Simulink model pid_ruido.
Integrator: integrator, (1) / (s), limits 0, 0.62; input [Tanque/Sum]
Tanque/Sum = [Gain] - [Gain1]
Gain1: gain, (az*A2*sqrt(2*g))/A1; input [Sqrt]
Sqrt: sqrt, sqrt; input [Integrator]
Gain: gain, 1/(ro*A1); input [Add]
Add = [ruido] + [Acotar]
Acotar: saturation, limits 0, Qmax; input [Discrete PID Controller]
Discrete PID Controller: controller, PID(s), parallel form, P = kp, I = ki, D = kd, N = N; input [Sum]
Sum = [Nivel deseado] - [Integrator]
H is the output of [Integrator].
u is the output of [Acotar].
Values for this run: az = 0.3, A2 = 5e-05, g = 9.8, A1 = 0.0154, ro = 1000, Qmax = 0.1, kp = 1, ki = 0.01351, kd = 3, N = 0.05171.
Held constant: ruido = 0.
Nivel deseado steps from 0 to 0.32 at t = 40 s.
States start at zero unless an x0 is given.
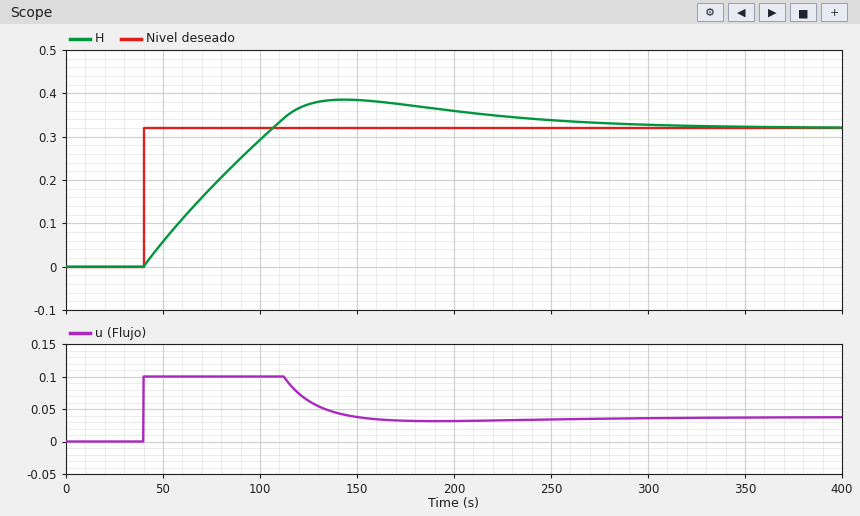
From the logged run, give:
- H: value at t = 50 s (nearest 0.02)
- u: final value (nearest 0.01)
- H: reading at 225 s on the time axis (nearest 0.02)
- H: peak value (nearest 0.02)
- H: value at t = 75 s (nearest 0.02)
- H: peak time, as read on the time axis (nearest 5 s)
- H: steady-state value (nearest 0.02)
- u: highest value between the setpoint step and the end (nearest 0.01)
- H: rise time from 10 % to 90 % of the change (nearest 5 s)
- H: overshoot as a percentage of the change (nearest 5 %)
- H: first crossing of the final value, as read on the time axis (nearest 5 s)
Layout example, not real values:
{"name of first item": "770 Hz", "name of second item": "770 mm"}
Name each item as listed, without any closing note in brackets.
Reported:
{"H: value at t = 50 s": "0.06", "u: final value": "0.04", "H: reading at 225 s on the time axis": "0.34", "H: peak value": "0.38", "H: value at t = 75 s": "0.18", "H: peak time, as read on the time axis": "145 s", "H: steady-state value": "0.32", "u: highest value between the setpoint step and the end": "0.10", "H: rise time from 10 % to 90 % of the change": "55 s", "H: overshoot as a percentage of the change": "20 %", "H: first crossing of the final value, as read on the time axis": "105 s"}
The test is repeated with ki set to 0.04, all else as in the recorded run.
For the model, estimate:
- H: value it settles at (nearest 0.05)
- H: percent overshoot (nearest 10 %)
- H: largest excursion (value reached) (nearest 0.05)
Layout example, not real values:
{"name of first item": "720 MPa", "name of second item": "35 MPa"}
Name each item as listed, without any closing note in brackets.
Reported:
{"H: value it settles at": "0.30", "H: percent overshoot": "50 %", "H: largest excursion (value reached)": "0.50"}
